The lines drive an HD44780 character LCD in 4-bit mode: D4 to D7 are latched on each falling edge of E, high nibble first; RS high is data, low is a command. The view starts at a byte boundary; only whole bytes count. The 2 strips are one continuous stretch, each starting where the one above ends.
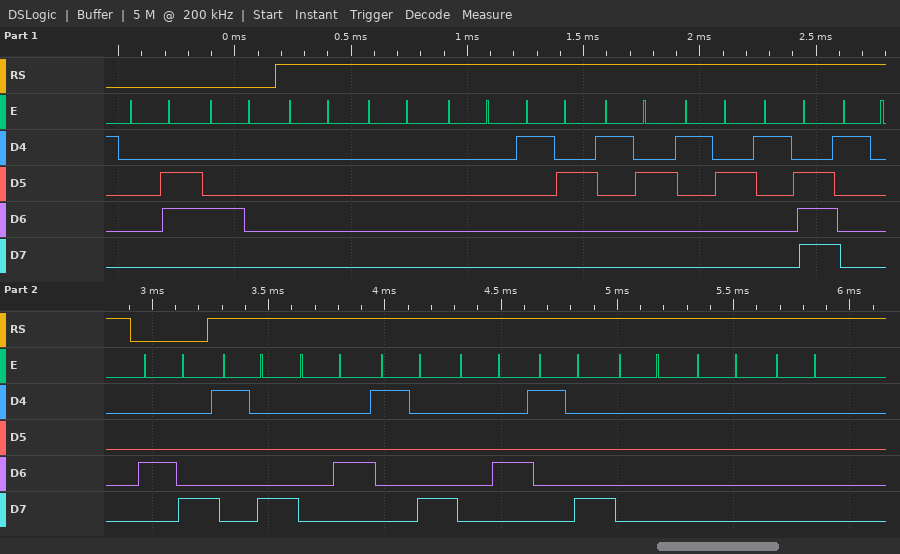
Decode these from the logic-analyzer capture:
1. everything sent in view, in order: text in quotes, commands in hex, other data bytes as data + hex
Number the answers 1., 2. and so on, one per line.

1. 0x06 0x40 data 00 00 00 12 12 12 1E 10 0x48 data 18 04 18 04 18 00 00 00
